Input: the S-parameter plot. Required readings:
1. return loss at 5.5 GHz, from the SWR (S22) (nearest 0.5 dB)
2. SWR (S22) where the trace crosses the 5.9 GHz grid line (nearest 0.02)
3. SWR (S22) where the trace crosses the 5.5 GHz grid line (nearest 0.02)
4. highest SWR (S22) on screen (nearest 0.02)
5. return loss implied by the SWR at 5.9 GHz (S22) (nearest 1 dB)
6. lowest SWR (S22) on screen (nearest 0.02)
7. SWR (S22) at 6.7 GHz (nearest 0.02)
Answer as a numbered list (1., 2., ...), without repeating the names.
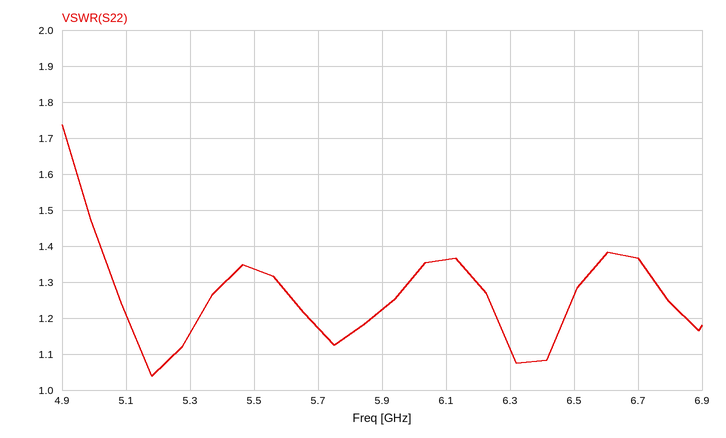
1. 17.0 dB
2. 1.22
3. 1.34
4. 1.74
5. 20 dB
6. 1.04
7. 1.36
